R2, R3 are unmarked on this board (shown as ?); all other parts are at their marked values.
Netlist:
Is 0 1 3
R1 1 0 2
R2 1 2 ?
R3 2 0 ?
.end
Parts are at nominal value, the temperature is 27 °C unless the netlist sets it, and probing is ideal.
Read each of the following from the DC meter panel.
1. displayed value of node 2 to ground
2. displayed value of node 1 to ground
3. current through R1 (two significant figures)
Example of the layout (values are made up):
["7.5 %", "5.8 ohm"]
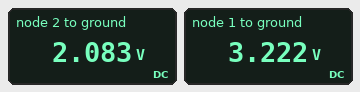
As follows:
["2.083 V", "3.222 V", "1.6 A"]
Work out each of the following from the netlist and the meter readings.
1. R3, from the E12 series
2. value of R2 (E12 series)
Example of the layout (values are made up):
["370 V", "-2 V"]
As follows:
["1.5 Ω", "0.82 Ω"]
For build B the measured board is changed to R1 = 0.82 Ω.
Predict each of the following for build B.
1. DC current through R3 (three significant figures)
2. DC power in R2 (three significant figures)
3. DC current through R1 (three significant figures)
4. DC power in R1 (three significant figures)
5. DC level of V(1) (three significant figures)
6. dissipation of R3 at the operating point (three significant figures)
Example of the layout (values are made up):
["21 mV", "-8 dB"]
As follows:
["783 mA", "503 mW", "2.22 A", "4.03 W", "1.82 V", "921 mW"]
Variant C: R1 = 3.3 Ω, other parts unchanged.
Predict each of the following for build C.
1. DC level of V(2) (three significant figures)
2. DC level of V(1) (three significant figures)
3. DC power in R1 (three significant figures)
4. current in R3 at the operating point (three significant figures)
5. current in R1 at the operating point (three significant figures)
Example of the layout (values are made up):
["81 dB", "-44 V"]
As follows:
["2.64 V", "4.09 V", "5.06 W", "1.76 A", "1.24 A"]
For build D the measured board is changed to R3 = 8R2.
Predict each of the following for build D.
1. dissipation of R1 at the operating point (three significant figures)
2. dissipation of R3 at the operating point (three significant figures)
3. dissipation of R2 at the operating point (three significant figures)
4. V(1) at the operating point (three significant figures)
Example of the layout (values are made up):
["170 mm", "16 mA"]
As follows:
["12.1 W", "2.43 W", "243 mW", "4.91 V"]
